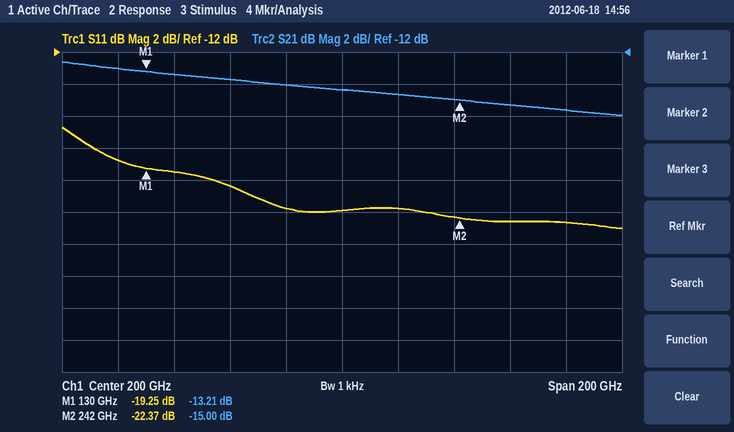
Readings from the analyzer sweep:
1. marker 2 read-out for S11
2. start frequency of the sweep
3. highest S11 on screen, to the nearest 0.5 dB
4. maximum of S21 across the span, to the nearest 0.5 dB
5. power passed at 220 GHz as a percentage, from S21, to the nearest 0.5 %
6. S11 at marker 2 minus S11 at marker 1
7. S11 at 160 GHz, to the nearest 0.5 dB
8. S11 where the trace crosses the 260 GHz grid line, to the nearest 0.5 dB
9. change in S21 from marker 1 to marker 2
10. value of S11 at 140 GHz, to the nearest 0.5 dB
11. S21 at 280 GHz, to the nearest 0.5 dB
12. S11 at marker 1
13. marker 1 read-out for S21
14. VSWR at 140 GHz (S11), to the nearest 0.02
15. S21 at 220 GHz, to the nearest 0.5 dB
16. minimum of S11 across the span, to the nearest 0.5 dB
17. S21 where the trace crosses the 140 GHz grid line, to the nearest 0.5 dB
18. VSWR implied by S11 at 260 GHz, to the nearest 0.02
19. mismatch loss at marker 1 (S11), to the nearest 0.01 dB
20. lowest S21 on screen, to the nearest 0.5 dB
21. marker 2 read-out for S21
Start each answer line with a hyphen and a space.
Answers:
- -22.37 dB
- 100 GHz
- -16.5 dB
- -12.5 dB
- 3.5 %
- -3.12 dB
- -20.5 dB
- -22.5 dB
- -1.79 dB
- -19.5 dB
- -15.5 dB
- -19.25 dB
- -13.21 dB
- 1.24
- -14.5 dB
- -23.0 dB
- -13.5 dB
- 1.16
- 0.05 dB
- -16.0 dB
- -15.00 dB
